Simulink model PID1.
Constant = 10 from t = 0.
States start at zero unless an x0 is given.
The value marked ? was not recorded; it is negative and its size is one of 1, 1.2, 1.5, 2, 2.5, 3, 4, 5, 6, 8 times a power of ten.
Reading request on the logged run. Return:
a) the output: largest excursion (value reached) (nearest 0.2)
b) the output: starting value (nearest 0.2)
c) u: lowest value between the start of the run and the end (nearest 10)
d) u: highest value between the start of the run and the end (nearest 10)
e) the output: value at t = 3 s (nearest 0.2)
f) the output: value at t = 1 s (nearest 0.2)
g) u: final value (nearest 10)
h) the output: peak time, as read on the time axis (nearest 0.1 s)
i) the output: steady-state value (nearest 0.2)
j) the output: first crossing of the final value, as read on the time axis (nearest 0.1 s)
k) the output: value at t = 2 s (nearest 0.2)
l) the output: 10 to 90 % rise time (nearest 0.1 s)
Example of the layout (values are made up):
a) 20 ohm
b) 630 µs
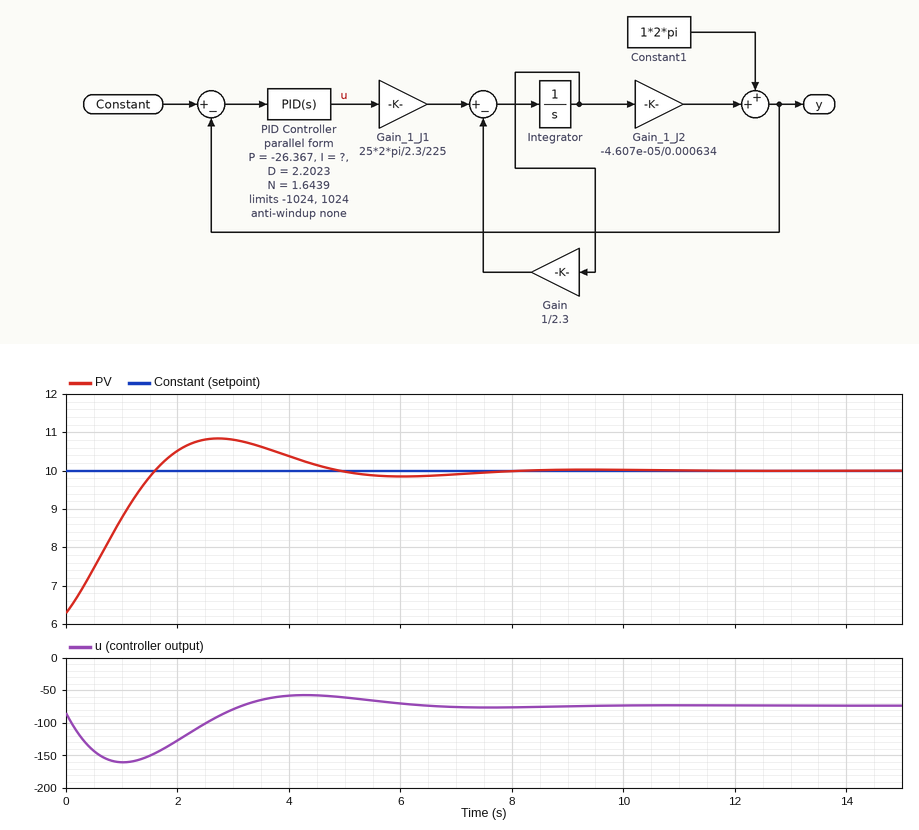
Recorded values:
a) 10.8
b) 6.2
c) -160
d) -60
e) 10.8
f) 8.8
g) -70
h) 2.7 s
i) 10.0
j) 1.6 s
k) 10.6
l) 1.2 s
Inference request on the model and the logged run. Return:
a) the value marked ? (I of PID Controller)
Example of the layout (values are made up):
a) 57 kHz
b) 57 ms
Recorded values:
a) -50
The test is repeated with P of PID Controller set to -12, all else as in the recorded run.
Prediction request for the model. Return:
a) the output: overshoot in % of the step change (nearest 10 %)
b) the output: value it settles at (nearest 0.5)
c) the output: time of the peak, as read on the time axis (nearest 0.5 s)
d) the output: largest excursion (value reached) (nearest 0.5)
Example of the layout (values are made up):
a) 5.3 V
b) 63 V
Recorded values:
a) 40 %
b) 10.0
c) 3.0 s
d) 11.5
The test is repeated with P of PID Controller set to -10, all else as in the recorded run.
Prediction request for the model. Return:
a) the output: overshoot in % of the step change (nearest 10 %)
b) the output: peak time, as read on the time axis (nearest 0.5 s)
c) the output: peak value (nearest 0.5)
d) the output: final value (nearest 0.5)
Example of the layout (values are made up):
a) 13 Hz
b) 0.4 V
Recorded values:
a) 40 %
b) 3.0 s
c) 11.5
d) 10.0
